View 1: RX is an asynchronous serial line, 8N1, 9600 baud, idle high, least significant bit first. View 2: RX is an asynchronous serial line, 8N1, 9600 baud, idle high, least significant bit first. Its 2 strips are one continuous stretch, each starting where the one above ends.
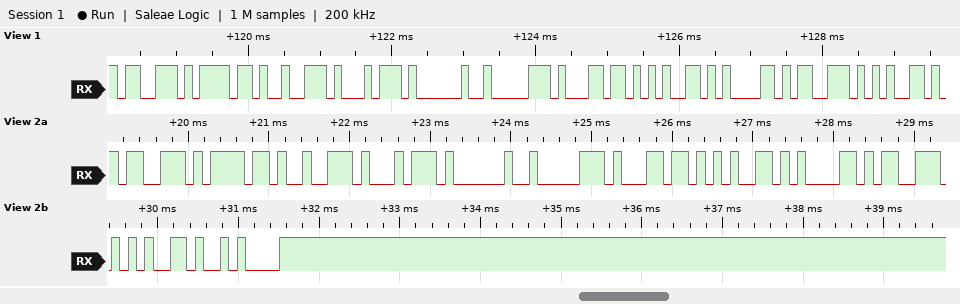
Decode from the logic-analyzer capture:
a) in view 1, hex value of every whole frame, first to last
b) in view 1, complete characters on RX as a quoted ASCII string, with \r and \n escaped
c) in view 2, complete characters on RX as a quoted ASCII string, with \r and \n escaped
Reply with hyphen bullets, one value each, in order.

- 0x73 0x6F 0x72 0x74 0x20 0x70 0x6C 0x65 0x61 0x73 0x65
- "sort please"
- "sort please\n"
